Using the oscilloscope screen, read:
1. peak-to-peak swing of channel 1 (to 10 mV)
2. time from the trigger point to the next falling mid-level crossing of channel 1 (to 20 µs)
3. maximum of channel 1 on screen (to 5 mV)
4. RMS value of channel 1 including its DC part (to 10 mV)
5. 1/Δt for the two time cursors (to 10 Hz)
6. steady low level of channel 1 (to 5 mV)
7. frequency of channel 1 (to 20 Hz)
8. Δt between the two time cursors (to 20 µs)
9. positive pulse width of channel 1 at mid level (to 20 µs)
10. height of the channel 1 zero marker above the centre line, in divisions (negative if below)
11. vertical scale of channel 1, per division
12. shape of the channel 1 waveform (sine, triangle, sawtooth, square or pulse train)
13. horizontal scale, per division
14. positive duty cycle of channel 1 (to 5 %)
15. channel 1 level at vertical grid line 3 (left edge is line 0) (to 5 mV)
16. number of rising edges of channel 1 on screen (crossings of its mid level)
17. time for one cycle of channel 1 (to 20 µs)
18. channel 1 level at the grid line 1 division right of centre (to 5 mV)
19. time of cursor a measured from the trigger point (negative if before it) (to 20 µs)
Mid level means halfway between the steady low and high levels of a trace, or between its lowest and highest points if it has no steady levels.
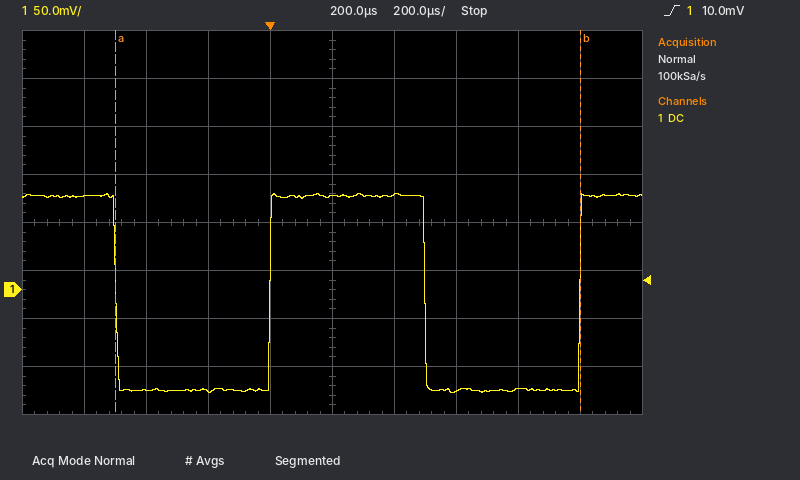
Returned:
210 mV
500 µs
100 mV
100 mV
670 Hz
-105 mV
1.00 kHz
1.50 ms
500 µs
-1.4 div
50 mV
square
200 µs
50 %
-105 mV
2
1.00 ms
100 mV
-500 µs
